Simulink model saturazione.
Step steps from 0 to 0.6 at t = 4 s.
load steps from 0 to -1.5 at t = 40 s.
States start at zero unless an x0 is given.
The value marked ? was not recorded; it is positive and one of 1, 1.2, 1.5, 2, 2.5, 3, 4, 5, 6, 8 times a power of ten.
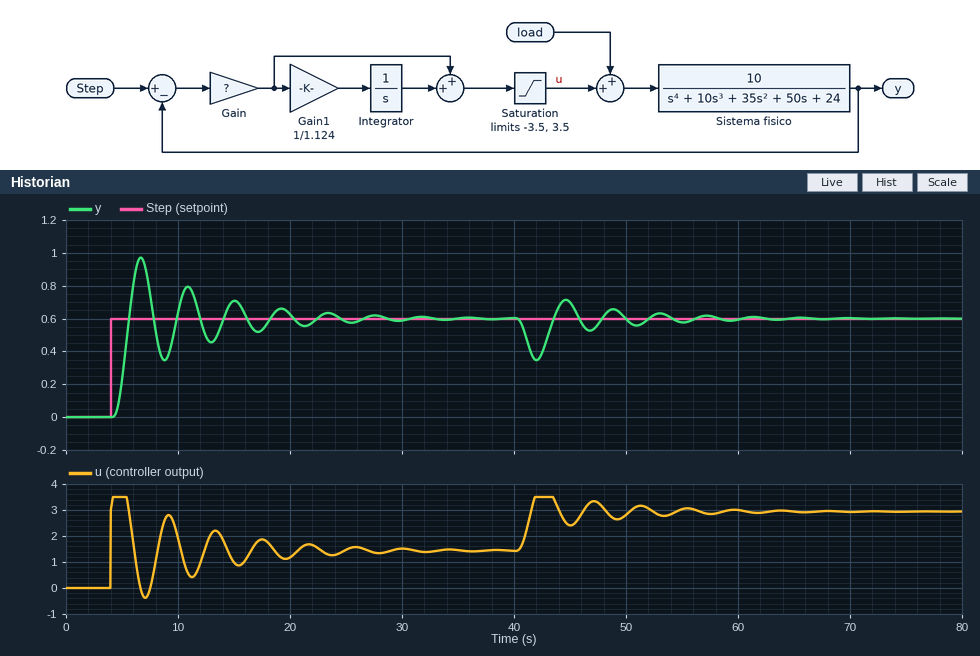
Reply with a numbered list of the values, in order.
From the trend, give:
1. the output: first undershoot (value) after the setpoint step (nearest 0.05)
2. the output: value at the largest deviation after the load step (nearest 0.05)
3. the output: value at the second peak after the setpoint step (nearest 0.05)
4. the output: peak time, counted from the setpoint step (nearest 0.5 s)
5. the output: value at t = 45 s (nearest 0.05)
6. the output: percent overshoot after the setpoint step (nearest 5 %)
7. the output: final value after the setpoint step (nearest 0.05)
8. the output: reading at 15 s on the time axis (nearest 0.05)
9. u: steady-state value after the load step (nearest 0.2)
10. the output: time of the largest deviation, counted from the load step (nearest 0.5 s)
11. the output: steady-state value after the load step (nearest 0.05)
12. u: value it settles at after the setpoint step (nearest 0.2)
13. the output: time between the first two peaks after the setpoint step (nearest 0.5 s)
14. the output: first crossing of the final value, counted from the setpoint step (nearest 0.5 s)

1. 0.35
2. 0.35
3. 0.80
4. 2.5 s
5. 0.70
6. 60 %
7. 0.60
8. 0.70
9. 3.0
10. 2.0 s
11. 0.60
12. 1.4
13. 4.0 s
14. 1.5 s
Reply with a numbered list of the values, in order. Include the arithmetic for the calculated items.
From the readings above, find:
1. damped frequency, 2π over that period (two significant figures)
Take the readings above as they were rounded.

1. 2π / 4 = 1.6 rad/s
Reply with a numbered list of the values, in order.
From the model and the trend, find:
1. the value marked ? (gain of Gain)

1. 5
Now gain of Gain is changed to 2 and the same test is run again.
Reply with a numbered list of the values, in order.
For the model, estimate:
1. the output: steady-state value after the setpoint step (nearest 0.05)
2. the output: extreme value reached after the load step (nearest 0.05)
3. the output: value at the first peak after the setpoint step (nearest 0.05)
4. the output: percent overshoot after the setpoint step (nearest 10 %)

1. 0.60
2. 0.25
3. 0.70
4. 20 %
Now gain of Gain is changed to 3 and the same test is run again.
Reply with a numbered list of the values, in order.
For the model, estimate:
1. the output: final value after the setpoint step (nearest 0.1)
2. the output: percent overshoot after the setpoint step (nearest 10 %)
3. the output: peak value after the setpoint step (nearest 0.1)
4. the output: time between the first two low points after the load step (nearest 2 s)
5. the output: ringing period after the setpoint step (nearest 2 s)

1. 0.6
2. 40 %
3. 0.8
4. 6 s
5. 6 s
